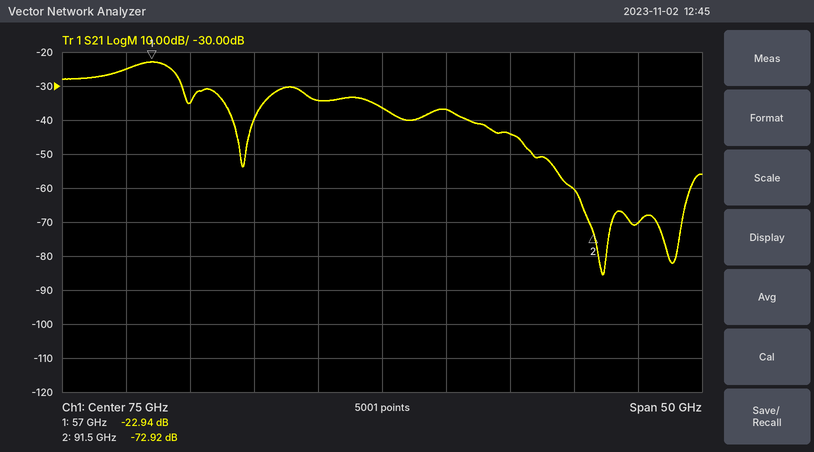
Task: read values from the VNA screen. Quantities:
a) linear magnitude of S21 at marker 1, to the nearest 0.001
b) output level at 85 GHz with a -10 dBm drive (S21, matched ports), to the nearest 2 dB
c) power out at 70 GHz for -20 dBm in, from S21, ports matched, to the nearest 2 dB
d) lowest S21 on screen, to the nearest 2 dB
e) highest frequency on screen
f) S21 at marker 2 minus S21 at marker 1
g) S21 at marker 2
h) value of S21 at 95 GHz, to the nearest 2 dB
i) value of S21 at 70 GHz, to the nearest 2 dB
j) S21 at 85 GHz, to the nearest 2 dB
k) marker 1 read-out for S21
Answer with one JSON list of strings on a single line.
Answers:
["0.071", "-54 dBm", "-54 dBm", "-86 dB", "100 GHz", "-49.98 dB", "-72.92 dB", "-70 dB", "-34 dB", "-44 dB", "-22.94 dB"]
